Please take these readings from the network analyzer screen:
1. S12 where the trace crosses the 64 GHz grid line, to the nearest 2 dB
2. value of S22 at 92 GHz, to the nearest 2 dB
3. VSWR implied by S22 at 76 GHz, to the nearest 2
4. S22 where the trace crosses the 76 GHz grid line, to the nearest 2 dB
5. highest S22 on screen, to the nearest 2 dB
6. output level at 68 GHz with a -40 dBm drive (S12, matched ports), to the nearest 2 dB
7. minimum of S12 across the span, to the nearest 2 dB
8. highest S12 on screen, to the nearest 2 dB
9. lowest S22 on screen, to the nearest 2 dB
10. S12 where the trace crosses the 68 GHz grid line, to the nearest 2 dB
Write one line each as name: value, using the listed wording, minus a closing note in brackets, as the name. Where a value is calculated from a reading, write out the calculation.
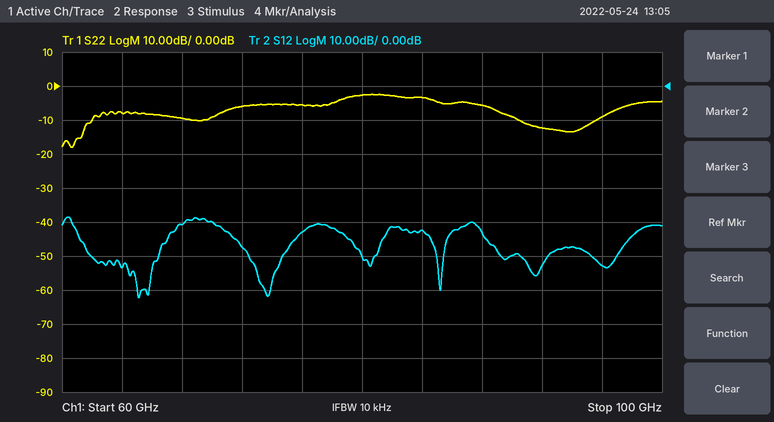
S12 where the trace crosses the 64 GHz grid line, to the nearest 2 dB: -54 dB
value of S22 at 92 GHz, to the nearest 2 dB: -12 dB
VSWR implied by S22 at 76 GHz, to the nearest 2: |Γ| = 10^(-6/20) = 0.5012; VSWR = (1 + 0.5012)/(1 − 0.5012) ≈ 3.01, so 4 to the nearest 2
S22 where the trace crosses the 76 GHz grid line, to the nearest 2 dB: -6 dB
highest S22 on screen, to the nearest 2 dB: -2 dB
output level at 68 GHz with a -40 dBm drive (S12, matched ports), to the nearest 2 dB: -40 dBm + (-40 dB) = -80 dBm
minimum of S12 across the span, to the nearest 2 dB: -62 dB
highest S12 on screen, to the nearest 2 dB: -38 dB
lowest S22 on screen, to the nearest 2 dB: -18 dB
S12 where the trace crosses the 68 GHz grid line, to the nearest 2 dB: -40 dB
